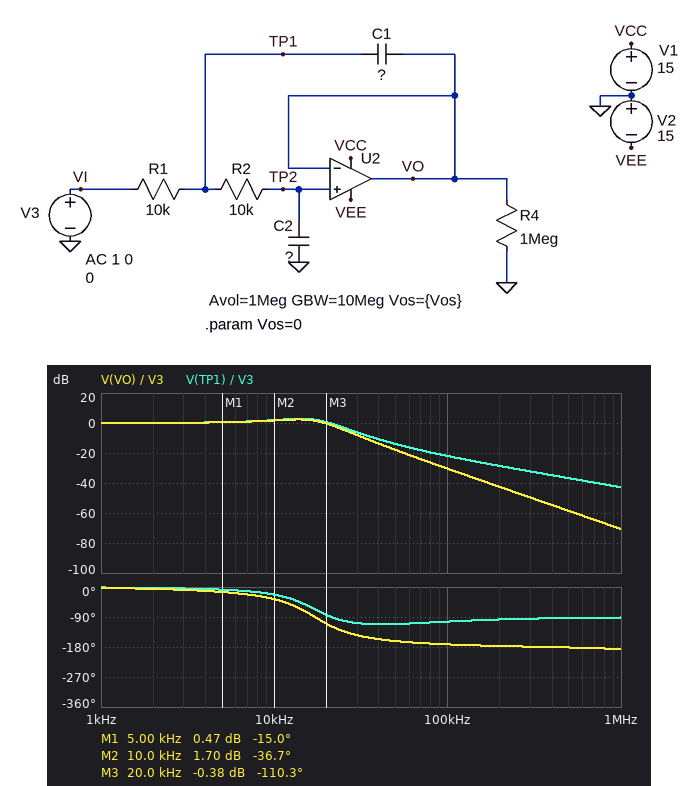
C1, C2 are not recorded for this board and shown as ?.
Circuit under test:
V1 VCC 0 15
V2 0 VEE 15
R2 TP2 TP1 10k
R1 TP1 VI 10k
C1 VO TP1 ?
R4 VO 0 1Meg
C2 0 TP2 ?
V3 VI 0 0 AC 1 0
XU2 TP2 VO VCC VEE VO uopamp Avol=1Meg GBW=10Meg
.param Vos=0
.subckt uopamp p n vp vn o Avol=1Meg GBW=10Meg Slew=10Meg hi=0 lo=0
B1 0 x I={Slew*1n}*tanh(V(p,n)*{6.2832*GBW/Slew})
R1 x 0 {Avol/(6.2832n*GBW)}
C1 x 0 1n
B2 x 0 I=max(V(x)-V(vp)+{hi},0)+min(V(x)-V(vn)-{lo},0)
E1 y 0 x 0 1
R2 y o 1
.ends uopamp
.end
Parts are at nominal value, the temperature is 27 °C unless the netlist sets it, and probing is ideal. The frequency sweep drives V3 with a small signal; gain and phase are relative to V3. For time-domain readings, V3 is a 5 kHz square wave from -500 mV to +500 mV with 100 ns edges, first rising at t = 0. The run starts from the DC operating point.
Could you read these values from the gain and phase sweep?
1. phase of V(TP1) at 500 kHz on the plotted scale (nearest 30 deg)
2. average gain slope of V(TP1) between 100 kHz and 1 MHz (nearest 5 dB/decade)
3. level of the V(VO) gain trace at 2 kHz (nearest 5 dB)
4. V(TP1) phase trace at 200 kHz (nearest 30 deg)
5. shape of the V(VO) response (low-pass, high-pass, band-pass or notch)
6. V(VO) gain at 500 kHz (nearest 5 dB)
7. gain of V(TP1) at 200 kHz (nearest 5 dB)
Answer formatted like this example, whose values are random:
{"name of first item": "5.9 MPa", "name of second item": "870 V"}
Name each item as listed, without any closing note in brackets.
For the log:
{"phase of V(TP1) at 500 kHz on the plotted scale": "-90 deg", "average gain slope of V(TP1) between 100 kHz and 1 MHz": "-20 dB/decade", "level of the V(VO) gain trace at 2 kHz": "0 dB", "V(TP1) phase trace at 200 kHz": "-90 deg", "shape of the V(VO) response": "low-pass", "V(VO) gain at 500 kHz": "-60 dB", "gain of V(TP1) at 200 kHz": "-30 dB"}
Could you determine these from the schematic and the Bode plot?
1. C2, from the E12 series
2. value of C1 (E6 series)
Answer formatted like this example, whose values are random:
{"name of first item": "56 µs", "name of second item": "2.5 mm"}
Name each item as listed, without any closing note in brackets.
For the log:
{"C2, from the E12 series": "390 pF", "value of C1": "2.2 nF"}
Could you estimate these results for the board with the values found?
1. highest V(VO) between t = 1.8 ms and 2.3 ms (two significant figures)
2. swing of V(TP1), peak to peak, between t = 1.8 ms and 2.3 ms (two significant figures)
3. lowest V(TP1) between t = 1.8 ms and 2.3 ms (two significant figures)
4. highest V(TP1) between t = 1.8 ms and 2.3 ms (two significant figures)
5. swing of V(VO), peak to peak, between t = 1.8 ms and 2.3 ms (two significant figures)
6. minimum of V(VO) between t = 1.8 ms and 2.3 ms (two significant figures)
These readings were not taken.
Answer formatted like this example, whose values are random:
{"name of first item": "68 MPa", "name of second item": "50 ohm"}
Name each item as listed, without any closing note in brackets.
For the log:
{"highest V(VO) between t = 1.8 ms and 2.3 ms": "740 mV", "swing of V(TP1), peak to peak, between t = 1.8 ms and 2.3 ms": "1.5 V", "lowest V(TP1) between t = 1.8 ms and 2.3 ms": "-760 mV", "highest V(TP1) between t = 1.8 ms and 2.3 ms": "760 mV", "swing of V(VO), peak to peak, between t = 1.8 ms and 2.3 ms": "1.5 V", "minimum of V(VO) between t = 1.8 ms and 2.3 ms": "-740 mV"}
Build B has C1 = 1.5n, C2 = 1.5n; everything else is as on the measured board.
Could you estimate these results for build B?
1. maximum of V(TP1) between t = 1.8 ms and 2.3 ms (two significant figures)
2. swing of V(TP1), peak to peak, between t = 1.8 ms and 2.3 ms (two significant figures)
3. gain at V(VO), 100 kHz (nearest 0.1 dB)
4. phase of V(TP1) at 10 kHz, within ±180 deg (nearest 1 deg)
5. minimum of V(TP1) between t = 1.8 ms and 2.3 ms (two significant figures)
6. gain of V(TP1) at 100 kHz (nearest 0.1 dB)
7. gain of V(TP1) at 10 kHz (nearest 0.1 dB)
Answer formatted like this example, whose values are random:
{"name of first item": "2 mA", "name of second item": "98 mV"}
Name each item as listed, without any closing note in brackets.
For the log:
{"maximum of V(TP1) between t = 1.8 ms and 2.3 ms": "500 mV", "swing of V(TP1), peak to peak, between t = 1.8 ms and 2.3 ms": "1.0 V", "gain at V(VO), 100 kHz": "-39.1 dB", "phase of V(TP1) at 10 kHz, within ±180 deg": "-43 deg", "minimum of V(TP1) between t = 1.8 ms and 2.3 ms": "-500 mV", "gain of V(TP1) at 100 kHz": "-19.5 dB", "gain of V(TP1) at 10 kHz": "-2.8 dB"}
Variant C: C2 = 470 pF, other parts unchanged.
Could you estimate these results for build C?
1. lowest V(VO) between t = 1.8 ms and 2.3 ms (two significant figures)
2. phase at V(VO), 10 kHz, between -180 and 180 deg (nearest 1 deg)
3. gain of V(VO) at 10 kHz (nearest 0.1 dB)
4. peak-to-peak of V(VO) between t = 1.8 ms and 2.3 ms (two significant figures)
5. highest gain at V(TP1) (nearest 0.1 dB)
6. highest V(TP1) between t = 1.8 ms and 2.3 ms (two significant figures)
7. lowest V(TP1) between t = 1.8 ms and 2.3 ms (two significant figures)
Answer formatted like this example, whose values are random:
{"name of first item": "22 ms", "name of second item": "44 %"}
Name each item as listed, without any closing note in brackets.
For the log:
{"lowest V(VO) between t = 1.8 ms and 2.3 ms": "-700 mV", "phase at V(VO), 10 kHz, between -180 and 180 deg": "-45 deg", "gain of V(VO) at 10 kHz": "1.6 dB", "peak-to-peak of V(VO) between t = 1.8 ms and 2.3 ms": "1.4 V", "highest gain at V(TP1)": "2.3 dB", "highest V(TP1) between t = 1.8 ms and 2.3 ms": "720 mV", "lowest V(TP1) between t = 1.8 ms and 2.3 ms": "-720 mV"}
